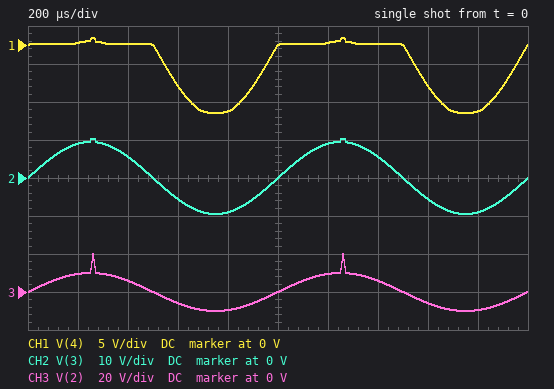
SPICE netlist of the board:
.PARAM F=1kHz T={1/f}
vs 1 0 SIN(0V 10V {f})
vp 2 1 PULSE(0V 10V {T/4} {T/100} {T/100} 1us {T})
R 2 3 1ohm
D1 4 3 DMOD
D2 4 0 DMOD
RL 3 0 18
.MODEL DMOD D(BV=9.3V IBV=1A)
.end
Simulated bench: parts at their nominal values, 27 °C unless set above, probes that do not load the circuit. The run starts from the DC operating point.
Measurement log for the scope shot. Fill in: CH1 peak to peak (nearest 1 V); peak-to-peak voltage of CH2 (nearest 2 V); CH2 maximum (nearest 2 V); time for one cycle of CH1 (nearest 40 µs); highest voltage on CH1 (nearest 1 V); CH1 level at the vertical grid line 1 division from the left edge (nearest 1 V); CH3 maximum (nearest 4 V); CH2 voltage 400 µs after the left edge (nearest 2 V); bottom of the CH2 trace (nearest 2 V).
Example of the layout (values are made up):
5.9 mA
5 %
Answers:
10 V
20 V
10 V
1.00 ms
1 V
0 V
20 V
6 V
-10 V
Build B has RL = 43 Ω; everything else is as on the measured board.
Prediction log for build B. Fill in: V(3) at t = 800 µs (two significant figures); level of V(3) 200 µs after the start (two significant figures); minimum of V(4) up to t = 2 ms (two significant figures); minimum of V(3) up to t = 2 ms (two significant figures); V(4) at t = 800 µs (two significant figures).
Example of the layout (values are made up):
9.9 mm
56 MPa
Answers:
-9.3 V
9.3 V
-9.1 V
-9.8 V
-8.9 V
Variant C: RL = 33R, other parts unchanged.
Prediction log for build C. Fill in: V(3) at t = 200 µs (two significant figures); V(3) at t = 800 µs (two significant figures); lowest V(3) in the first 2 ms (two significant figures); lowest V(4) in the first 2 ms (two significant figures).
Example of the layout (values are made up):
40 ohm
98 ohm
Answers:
9.2 V
-9.2 V
-9.7 V
-9.1 V
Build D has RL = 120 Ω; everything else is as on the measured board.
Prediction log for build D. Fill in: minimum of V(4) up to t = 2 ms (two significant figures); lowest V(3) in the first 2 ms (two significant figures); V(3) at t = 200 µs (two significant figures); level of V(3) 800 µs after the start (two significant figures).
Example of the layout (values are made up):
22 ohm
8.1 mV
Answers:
-9.2 V
-9.9 V
9.4 V
-9.4 V
